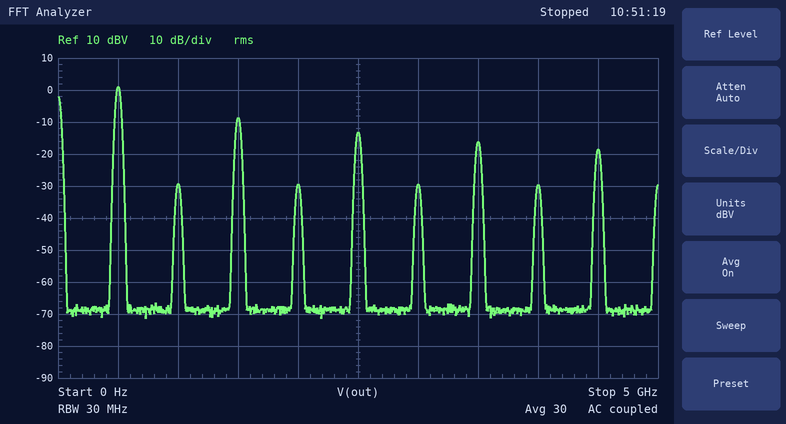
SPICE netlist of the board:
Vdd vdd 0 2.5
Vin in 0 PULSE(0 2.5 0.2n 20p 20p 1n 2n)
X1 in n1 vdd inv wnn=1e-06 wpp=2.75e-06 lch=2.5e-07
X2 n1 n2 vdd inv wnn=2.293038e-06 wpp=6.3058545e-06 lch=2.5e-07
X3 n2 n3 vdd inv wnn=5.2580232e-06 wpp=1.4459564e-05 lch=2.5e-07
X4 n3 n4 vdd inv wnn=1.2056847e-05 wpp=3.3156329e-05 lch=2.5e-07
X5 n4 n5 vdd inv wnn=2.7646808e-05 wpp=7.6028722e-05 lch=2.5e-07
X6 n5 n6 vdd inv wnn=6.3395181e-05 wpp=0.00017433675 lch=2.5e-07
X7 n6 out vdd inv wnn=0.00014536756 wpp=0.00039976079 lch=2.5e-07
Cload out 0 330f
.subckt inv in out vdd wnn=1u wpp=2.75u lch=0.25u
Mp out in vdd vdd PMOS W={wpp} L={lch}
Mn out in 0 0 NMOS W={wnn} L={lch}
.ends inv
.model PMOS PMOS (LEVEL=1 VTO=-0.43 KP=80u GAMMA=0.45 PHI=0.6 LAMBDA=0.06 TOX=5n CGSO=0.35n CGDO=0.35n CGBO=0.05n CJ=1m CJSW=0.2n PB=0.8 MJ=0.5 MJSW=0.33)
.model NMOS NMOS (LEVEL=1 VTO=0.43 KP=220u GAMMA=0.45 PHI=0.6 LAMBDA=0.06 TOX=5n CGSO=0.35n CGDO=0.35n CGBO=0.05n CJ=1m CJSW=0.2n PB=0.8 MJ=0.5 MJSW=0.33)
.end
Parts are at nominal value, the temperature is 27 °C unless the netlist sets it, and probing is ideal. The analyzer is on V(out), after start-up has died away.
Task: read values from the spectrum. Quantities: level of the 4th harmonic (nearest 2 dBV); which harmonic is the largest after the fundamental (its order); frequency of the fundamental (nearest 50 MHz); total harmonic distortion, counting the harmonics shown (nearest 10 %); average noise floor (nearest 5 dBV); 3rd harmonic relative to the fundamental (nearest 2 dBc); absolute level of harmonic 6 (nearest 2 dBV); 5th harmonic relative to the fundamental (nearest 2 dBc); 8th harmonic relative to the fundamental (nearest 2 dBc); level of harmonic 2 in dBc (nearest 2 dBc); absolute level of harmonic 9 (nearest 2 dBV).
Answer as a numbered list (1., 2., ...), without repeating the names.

1. -30 dBV
2. 3
3. 500 MHz
4. 40 %
5. -70 dBV
6. -10 dBc
7. -30 dBV
8. -14 dBc
9. -30 dBc
10. -30 dBc
11. -18 dBV
